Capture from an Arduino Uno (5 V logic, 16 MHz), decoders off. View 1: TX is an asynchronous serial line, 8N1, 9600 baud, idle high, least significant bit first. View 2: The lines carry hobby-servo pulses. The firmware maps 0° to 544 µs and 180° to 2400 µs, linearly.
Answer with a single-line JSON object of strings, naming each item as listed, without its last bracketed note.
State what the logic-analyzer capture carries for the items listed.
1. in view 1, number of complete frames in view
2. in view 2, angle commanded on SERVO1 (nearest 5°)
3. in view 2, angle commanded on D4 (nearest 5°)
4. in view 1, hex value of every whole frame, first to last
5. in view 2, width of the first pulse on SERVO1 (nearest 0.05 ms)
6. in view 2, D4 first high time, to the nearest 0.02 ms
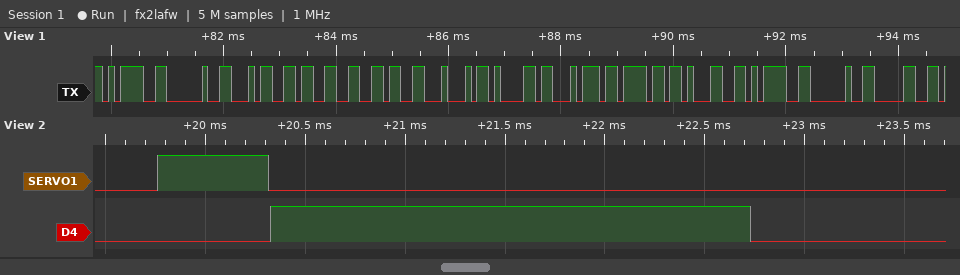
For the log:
{"in view 1, number of complete frames in view": "13", "in view 2, angle commanded on SERVO1": "0°", "in view 2, angle commanded on D4": "180°", "in view 1, hex value of every whole frame, first to last": "3D 20 34 33 36 44 61 74 6F 31 3D 20 30", "in view 2, width of the first pulse on SERVO1": "0.55 ms", "in view 2, D4 first high time, to the nearest 0.02 ms": "2.40 ms"}
